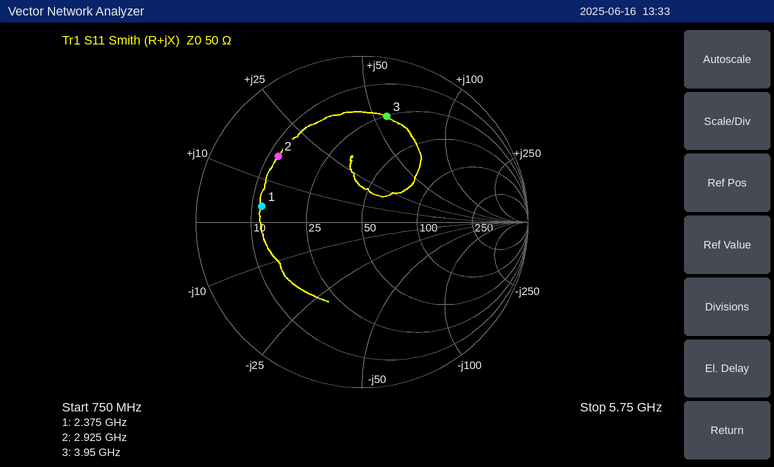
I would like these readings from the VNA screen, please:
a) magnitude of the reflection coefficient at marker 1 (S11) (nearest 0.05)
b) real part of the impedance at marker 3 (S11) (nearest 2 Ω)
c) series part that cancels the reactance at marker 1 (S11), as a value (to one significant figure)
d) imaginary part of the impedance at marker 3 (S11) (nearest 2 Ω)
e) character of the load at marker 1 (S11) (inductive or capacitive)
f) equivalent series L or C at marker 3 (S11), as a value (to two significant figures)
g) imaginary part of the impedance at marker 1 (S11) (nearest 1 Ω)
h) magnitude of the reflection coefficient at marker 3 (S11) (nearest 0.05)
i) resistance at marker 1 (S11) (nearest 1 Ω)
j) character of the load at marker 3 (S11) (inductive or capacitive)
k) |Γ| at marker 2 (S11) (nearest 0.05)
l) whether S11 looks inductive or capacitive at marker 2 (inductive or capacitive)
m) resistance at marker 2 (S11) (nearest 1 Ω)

0.60
26 Ω
20 pF
+56 Ω
inductive
2.3 nH
+4 Ω
0.65
12 Ω
inductive
0.65
inductive
12 Ω
